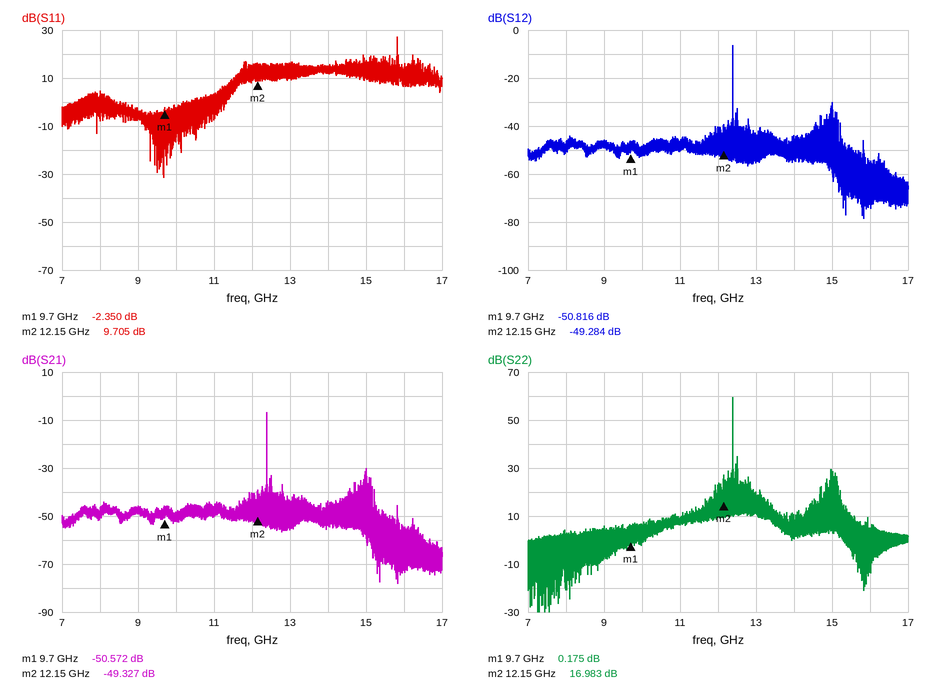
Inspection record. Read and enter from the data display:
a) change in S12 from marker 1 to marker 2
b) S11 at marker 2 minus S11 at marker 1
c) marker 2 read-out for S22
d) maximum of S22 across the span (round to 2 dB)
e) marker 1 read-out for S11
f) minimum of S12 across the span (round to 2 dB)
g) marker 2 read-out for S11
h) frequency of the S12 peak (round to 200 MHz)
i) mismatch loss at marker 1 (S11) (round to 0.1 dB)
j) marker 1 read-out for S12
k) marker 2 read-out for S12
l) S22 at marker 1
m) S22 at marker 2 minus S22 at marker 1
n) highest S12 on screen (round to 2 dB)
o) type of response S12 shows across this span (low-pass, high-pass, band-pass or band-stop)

1.532 dB
12.055 dB
16.983 dB
60 dB
-2.350 dB
-78 dB
9.705 dB
12.4 GHz
3.8 dB
-50.816 dB
-49.284 dB
0.175 dB
16.808 dB
-6 dB
band-pass
